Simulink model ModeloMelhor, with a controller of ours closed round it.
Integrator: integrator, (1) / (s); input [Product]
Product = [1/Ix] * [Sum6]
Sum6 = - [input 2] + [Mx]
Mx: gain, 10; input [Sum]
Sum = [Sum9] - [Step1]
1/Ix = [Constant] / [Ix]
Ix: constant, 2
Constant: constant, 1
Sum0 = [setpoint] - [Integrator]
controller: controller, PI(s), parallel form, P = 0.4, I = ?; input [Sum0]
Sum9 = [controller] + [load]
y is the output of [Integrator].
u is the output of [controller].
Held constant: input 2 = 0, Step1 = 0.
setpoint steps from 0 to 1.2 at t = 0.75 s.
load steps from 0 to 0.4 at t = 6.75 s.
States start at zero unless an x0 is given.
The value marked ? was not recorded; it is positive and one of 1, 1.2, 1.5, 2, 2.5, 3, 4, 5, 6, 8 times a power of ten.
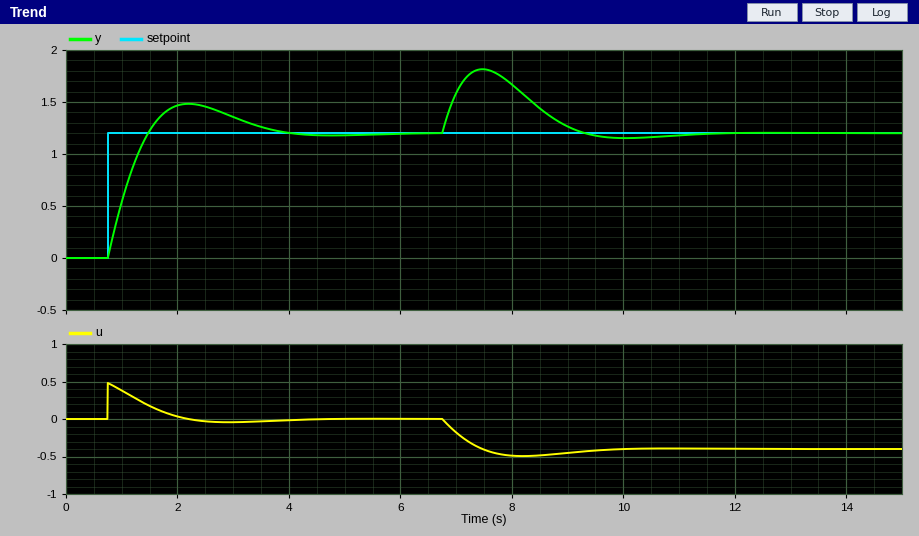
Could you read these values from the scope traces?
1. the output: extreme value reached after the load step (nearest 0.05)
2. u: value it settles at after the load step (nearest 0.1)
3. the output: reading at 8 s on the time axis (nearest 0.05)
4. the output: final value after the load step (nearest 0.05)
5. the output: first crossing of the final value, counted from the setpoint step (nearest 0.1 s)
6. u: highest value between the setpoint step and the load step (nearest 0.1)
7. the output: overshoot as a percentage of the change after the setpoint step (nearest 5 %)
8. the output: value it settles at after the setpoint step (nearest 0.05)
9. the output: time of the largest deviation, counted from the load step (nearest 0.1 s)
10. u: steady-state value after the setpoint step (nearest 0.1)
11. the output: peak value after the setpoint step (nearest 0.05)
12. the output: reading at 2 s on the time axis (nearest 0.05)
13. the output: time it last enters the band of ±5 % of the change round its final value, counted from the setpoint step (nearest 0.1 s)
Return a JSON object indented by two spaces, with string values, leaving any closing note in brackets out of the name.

{
  "the output: extreme value reached after the load step": "1.80",
  "u: value it settles at after the load step": "-0.4",
  "the output: reading at 8 s on the time axis": "1.65",
  "the output: final value after the load step": "1.20",
  "the output: first crossing of the final value, counted from the setpoint step": "0.7 s",
  "u: highest value between the setpoint step and the load step": "0.5",
  "the output: overshoot as a percentage of the change after the setpoint step": "25 %",
  "the output: value it settles at after the setpoint step": "1.20",
  "the output: time of the largest deviation, counted from the load step": "0.7 s",
  "u: steady-state value after the setpoint step": "0.0",
  "the output: peak value after the setpoint step": "1.50",
  "the output: reading at 2 s on the time axis": "1.45",
  "the output: time it last enters the band of ±5 % of the change round its final value, counted from the setpoint step": "2.8 s"
}
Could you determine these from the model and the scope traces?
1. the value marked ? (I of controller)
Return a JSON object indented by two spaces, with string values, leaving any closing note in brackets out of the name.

{
  "the value marked ?": "0.5"
}
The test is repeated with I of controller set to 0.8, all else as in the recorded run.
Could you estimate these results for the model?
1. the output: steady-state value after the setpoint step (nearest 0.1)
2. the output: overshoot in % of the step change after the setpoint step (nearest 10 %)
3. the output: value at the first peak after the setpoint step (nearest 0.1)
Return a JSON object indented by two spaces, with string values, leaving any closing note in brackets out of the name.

{
  "the output: steady-state value after the setpoint step": "1.2",
  "the output: overshoot in % of the step change after the setpoint step": "30 %",
  "the output: value at the first peak after the setpoint step": "1.6"
}
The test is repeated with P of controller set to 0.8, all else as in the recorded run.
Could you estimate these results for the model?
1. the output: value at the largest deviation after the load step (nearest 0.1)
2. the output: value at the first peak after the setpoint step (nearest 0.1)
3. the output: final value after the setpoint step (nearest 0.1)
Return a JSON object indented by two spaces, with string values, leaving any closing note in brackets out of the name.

{
  "the output: value at the largest deviation after the load step": "1.6",
  "the output: value at the first peak after the setpoint step": "1.3",
  "the output: final value after the setpoint step": "1.2"
}
